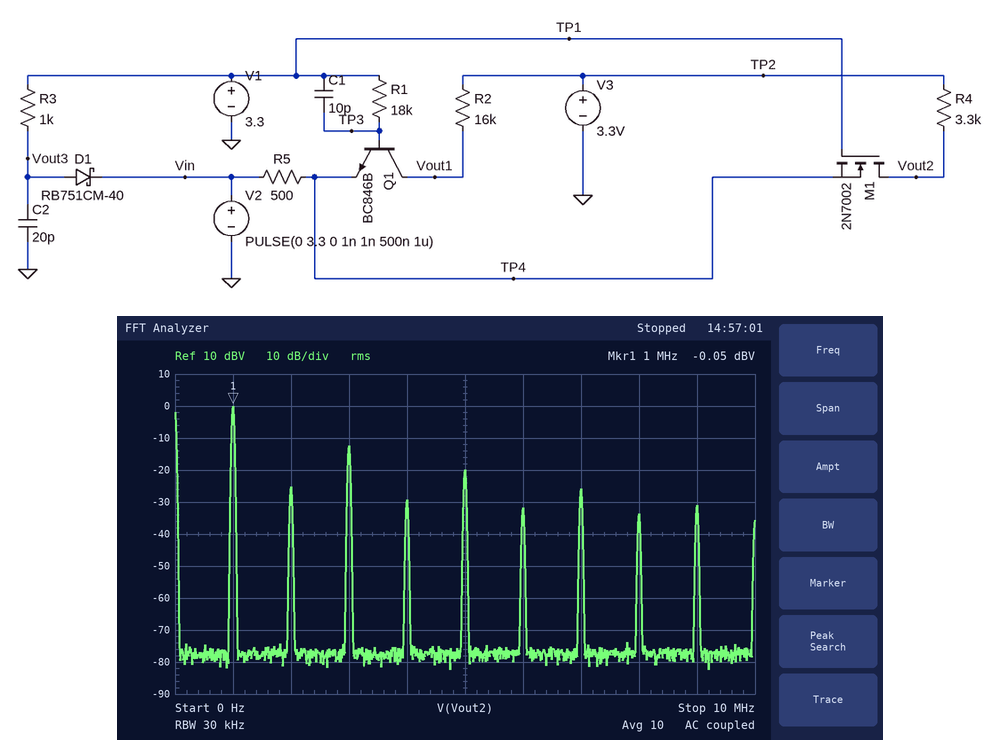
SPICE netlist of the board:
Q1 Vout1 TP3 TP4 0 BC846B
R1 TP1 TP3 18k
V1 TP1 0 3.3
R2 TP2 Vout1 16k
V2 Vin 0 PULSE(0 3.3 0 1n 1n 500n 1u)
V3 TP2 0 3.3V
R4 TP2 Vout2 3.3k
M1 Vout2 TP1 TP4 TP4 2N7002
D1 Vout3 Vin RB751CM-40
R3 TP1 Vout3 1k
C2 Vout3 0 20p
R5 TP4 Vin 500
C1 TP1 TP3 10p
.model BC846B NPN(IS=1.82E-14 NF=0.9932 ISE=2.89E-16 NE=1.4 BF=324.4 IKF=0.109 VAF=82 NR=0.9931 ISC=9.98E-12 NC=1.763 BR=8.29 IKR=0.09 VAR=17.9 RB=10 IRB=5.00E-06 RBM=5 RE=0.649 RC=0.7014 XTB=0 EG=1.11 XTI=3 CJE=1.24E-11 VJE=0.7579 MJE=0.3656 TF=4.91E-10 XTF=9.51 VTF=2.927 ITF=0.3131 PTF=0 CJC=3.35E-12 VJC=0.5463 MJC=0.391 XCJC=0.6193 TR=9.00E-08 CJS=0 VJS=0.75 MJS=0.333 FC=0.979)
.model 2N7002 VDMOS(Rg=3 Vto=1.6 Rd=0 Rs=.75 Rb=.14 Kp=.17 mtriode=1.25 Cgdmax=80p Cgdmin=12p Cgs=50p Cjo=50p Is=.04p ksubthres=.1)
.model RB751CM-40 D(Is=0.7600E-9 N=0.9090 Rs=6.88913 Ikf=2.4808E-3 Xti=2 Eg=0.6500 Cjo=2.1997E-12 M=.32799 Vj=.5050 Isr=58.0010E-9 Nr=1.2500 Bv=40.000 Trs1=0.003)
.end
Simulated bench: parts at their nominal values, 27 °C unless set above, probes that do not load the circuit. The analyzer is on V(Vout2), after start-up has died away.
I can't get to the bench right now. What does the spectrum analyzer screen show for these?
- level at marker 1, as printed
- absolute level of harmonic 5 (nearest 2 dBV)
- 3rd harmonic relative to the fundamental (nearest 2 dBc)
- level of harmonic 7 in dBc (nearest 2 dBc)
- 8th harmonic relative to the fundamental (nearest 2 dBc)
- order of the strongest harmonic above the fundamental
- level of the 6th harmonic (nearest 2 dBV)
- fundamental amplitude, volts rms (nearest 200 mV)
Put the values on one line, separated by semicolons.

-0.05 dBV; -20 dBV; -12 dBc; -26 dBc; -34 dBc; 3; -32 dBV; 1.0 V
